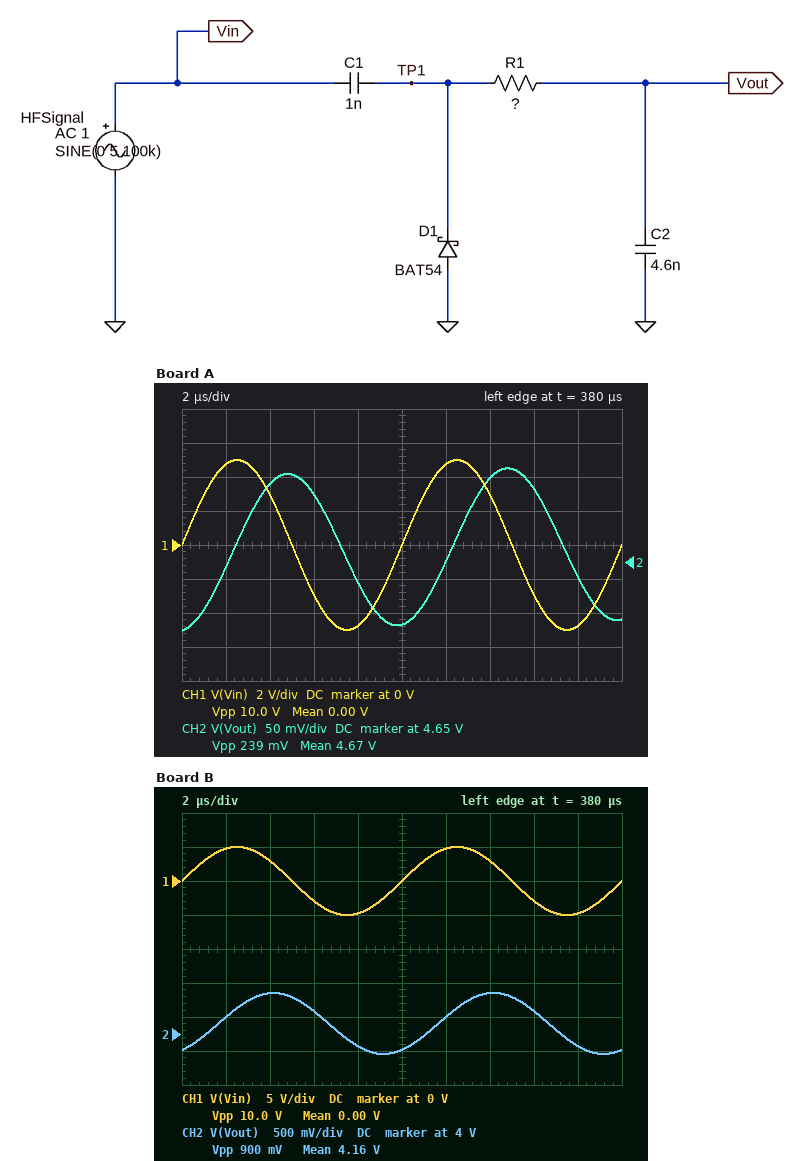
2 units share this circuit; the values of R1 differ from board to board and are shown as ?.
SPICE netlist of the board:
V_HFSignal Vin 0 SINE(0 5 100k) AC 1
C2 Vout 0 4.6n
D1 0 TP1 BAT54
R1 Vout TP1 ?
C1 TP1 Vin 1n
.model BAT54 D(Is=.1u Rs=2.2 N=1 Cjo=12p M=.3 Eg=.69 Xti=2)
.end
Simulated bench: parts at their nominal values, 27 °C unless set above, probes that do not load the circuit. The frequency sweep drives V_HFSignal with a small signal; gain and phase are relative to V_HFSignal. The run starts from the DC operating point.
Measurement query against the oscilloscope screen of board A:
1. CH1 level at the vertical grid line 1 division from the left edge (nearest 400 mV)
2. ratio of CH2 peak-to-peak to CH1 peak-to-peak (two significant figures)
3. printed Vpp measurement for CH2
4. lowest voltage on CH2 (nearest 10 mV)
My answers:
4.8 V
0.024
239 mV
4.55 V
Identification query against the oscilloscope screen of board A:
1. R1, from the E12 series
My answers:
15 kΩ
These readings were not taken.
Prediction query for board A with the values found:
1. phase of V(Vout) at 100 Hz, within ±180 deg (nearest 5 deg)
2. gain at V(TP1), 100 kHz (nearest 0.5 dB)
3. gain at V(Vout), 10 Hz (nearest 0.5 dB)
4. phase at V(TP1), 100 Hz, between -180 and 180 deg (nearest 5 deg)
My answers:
45 deg
0 dB
-36.0 dB
50 deg
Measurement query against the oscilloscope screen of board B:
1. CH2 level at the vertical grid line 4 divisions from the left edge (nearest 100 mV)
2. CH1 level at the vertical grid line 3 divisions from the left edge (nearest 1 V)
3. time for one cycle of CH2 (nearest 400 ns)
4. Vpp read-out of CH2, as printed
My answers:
3.8 V
-3 V
10.0 µs
900 mV
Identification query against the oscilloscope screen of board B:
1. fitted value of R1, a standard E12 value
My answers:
3.3 kΩ
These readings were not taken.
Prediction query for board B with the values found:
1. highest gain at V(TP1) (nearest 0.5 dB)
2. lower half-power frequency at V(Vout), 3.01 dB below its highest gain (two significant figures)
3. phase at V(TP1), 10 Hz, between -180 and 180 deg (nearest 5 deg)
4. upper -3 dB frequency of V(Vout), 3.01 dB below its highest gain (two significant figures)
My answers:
0 dB
110 Hz
85 deg
59 kHz
